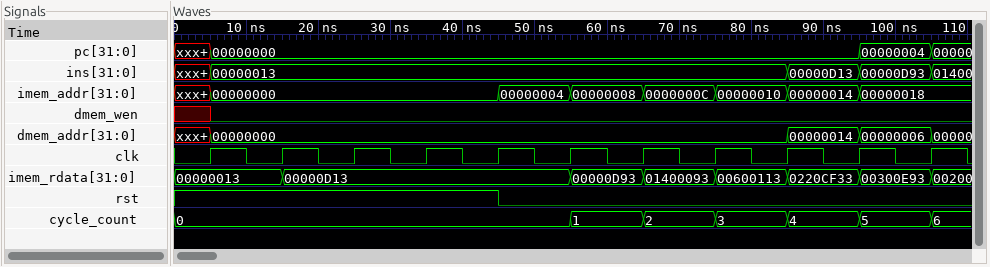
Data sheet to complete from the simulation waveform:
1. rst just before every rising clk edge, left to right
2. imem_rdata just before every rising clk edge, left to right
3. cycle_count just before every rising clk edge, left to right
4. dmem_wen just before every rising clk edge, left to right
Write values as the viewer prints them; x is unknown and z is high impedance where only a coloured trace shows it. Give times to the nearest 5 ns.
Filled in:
1 1 1 1 1 0 0 0 0 0 0
00000013, 00000013, 00000D13, 00000D13, 00000D13, 00000D13, 00000D93, 01400093, 00600113, 0220CF33, 00300E93
0, 0, 0, 0, 0, 0, 1, 2, 3, 4, 5
x 0 0 0 0 0 0 0 0 0 0
